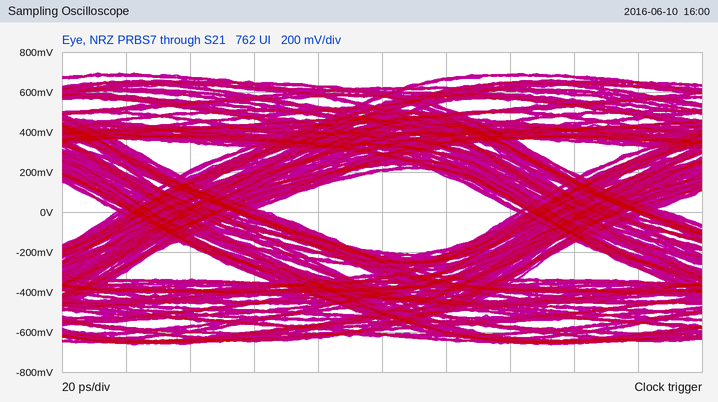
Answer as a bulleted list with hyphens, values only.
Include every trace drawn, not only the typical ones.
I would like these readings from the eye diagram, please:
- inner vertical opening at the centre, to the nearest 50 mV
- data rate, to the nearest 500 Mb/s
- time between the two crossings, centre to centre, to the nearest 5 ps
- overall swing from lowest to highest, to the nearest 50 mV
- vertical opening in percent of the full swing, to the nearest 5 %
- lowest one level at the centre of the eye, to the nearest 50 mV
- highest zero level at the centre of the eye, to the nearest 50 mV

- 400 mV
- 8.0 Gb/s
- 125 ps
- 1.35 V
- 30 %
- 200 mV
- -200 mV
